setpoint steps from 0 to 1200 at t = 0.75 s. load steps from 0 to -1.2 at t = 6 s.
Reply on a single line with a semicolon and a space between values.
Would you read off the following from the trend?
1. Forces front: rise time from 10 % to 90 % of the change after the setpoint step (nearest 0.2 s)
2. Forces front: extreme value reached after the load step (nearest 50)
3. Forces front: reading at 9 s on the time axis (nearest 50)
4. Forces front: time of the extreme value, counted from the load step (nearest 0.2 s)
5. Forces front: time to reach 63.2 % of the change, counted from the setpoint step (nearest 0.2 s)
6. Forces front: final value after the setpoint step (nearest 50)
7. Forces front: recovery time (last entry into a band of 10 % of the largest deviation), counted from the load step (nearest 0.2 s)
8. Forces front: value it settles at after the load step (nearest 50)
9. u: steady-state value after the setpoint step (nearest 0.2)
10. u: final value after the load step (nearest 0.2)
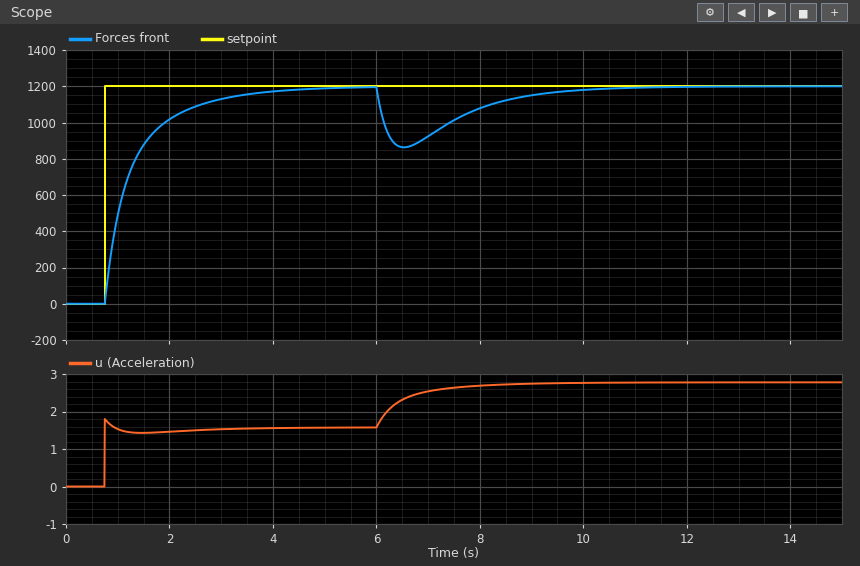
1.6 s; 850; 1150; 0.6 s; 0.6 s; 1200; 3.4 s; 1200; 1.6; 2.8
